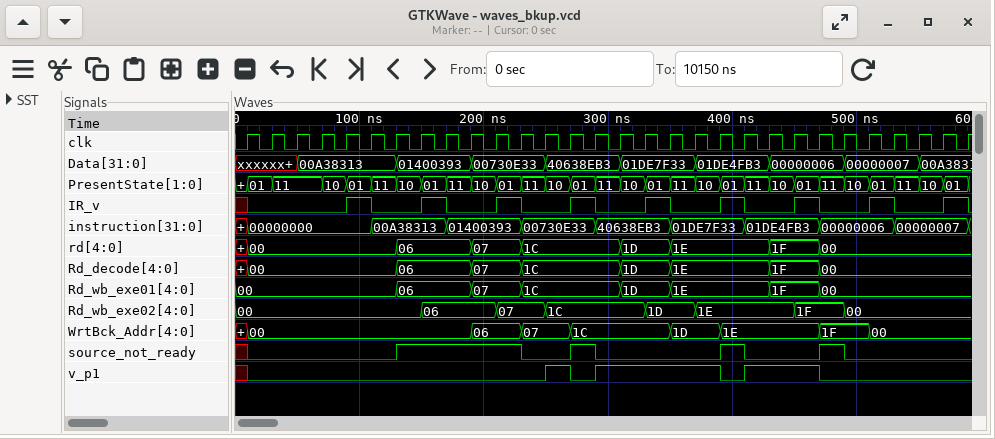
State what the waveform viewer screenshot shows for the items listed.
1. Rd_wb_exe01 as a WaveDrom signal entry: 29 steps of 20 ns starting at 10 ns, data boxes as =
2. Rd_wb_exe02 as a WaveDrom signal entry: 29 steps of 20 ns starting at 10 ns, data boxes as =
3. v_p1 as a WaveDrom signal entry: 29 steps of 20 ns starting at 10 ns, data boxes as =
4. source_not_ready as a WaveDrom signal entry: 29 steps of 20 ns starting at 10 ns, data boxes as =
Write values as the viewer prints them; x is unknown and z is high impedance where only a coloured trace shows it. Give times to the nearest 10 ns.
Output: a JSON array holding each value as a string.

["{name: 'Rd_wb_exe01', wave: '=.....=..=.=...=.=...=.=.....', data: '00 06 07 1C 1D 1E 1F 00'}", "{name: 'Rd_wb_exe02', wave: '=......=..=.=...=.=...=.=....', data: '00 06 07 1C 1D 1E 1F 00'}", "{name: 'v_p1', wave: '0...........101....01..0.....'}", "{name: 'source_not_ready', wave: '0.....1....0.10....10..10....'}"]
